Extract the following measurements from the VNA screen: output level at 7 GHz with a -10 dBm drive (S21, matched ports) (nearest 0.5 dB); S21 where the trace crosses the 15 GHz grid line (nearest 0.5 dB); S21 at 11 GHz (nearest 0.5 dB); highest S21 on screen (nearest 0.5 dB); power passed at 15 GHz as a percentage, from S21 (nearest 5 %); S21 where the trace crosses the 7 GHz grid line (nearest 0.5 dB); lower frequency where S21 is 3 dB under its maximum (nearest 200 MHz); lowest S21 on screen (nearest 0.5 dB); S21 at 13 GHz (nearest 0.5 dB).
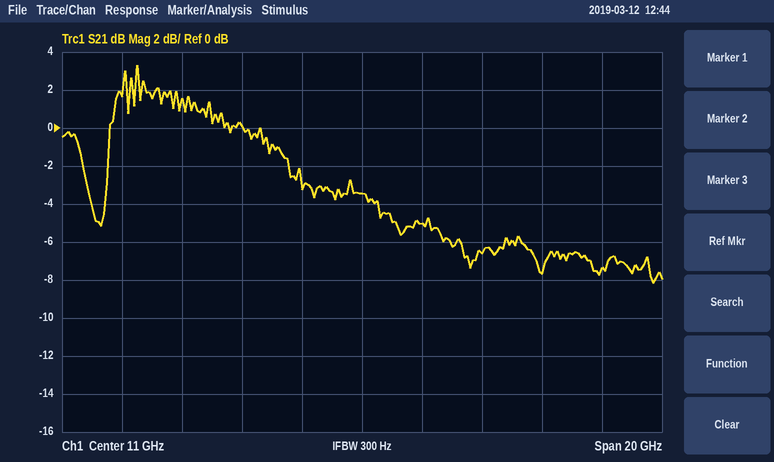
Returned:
-10.0 dBm
-6.5 dB
-3.5 dB
3.5 dB
20 %
0.0 dB
2.6 GHz
-8.0 dB
-5.0 dB
